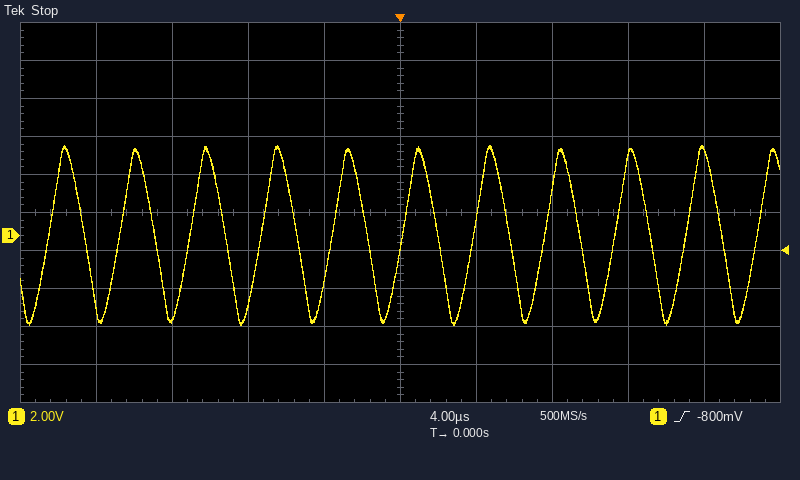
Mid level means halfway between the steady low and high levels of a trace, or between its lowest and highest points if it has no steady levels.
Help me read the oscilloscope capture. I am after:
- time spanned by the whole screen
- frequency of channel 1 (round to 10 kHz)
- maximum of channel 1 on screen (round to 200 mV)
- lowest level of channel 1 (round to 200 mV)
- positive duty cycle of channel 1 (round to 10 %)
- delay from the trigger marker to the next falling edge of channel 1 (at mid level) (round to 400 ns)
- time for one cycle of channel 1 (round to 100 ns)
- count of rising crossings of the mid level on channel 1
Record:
40 µs
270 kHz
4.8 V
-4.8 V
50 %
2.0 µs
3.7 µs
11
